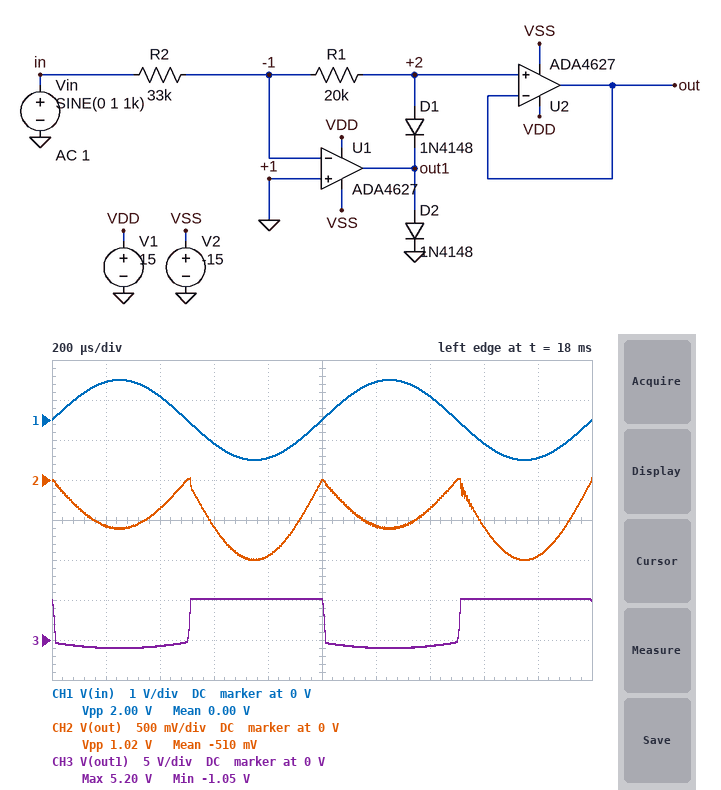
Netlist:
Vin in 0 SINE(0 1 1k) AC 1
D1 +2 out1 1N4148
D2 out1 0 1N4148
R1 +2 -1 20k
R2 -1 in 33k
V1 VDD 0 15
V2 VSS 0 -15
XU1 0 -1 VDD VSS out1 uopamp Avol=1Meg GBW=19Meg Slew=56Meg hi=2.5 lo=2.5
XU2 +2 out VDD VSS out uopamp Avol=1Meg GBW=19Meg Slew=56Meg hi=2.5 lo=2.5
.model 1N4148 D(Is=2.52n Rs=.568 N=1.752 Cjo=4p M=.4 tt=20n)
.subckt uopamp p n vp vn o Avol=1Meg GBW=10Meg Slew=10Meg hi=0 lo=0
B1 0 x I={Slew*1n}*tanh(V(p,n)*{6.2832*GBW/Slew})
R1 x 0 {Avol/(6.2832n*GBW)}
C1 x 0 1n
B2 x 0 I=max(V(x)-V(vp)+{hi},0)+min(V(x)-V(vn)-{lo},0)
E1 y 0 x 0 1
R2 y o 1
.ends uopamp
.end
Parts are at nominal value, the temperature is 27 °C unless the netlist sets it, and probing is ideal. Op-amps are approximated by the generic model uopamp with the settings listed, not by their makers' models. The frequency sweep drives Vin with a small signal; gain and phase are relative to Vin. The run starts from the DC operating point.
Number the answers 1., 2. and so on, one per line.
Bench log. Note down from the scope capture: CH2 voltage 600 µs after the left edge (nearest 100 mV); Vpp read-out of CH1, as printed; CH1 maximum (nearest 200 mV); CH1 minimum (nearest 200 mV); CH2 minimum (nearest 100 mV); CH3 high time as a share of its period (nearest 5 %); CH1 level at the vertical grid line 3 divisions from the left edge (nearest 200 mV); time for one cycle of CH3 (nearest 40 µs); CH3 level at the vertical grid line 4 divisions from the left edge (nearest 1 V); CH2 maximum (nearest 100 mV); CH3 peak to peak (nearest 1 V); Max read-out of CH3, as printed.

1. -600 mV
2. 2.00 V
3. 1.0 V
4. -1.0 V
5. -1.0 V
6. 50 %
7. -600 mV
8. 1.00 ms
9. 5 V
10. 0 V
11. 6 V
12. 5.20 V
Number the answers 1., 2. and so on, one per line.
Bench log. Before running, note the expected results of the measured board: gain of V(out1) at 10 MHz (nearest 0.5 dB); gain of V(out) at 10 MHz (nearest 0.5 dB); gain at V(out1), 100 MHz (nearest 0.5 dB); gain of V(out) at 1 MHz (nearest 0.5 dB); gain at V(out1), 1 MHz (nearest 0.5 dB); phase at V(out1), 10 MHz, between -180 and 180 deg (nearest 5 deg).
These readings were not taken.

1. -7.0 dB
2. -9.0 dB
3. -23.0 dB
4. -6.0 dB
5. 2.0 dB
6. 130 deg
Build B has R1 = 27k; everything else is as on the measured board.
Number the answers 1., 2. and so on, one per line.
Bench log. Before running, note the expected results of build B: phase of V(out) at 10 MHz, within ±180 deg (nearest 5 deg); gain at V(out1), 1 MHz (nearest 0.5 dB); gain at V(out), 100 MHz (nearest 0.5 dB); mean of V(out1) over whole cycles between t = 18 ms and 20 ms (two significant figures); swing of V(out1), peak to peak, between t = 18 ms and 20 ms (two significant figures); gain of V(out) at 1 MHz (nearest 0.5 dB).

1. 110 deg
2. 2.5 dB
3. -36.5 dB
4. 2.1 V
5. 6.4 V
6. -3.0 dB
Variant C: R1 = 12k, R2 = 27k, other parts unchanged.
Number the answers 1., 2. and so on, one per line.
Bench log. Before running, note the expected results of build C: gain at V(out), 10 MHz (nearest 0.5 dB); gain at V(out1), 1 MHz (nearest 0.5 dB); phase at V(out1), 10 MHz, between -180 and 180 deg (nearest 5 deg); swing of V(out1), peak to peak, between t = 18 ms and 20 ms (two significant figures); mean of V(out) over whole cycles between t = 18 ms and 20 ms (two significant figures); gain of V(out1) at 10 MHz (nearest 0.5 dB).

1. -12.0 dB
2. 3.0 dB
3. 125 deg
4. 6.1 V
5. -460 mV
6. -9.0 dB
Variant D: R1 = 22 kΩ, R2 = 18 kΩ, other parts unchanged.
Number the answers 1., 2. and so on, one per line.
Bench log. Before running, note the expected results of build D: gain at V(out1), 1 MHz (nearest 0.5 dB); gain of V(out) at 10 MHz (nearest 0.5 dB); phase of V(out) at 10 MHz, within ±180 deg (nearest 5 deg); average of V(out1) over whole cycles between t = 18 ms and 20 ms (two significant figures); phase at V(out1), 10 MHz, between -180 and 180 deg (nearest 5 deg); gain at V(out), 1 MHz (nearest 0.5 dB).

1. 7.0 dB
2. -4.5 dB
3. 105 deg
4. 2.0 V
5. 125 deg
6. 0 dB
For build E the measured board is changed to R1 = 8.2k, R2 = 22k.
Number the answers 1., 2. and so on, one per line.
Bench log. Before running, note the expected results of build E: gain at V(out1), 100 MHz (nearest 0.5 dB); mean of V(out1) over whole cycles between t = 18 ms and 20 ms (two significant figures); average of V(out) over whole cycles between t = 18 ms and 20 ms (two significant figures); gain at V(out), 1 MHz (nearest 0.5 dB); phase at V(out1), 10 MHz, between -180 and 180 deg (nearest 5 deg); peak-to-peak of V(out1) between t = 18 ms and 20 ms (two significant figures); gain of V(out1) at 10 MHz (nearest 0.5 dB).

1. -26.0 dB
2. 2.3 V
3. -440 mV
4. -12.0 dB
5. 120 deg
6. 6.0 V
7. -10.0 dB
